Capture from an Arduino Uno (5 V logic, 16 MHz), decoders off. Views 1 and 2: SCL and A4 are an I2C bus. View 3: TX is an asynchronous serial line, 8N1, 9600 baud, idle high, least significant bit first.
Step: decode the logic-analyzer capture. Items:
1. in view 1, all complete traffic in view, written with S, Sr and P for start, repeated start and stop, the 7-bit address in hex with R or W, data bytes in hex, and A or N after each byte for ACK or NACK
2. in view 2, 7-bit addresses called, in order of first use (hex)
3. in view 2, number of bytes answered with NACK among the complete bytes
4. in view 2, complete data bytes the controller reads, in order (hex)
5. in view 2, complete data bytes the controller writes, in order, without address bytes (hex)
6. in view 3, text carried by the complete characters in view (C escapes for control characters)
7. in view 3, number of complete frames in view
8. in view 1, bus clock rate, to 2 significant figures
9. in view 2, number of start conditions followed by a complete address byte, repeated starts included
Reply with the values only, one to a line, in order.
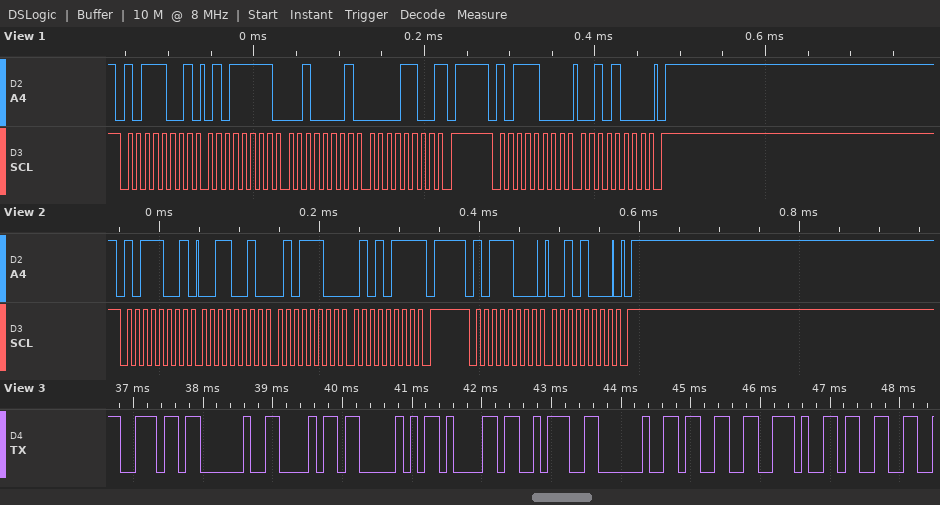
S 5CR A 5F A 21 A 0C N P S 5CW A 28 A P
0x5C
1
32 5C 57
28
"n hPa: 3.3"
10
100 kHz
2
